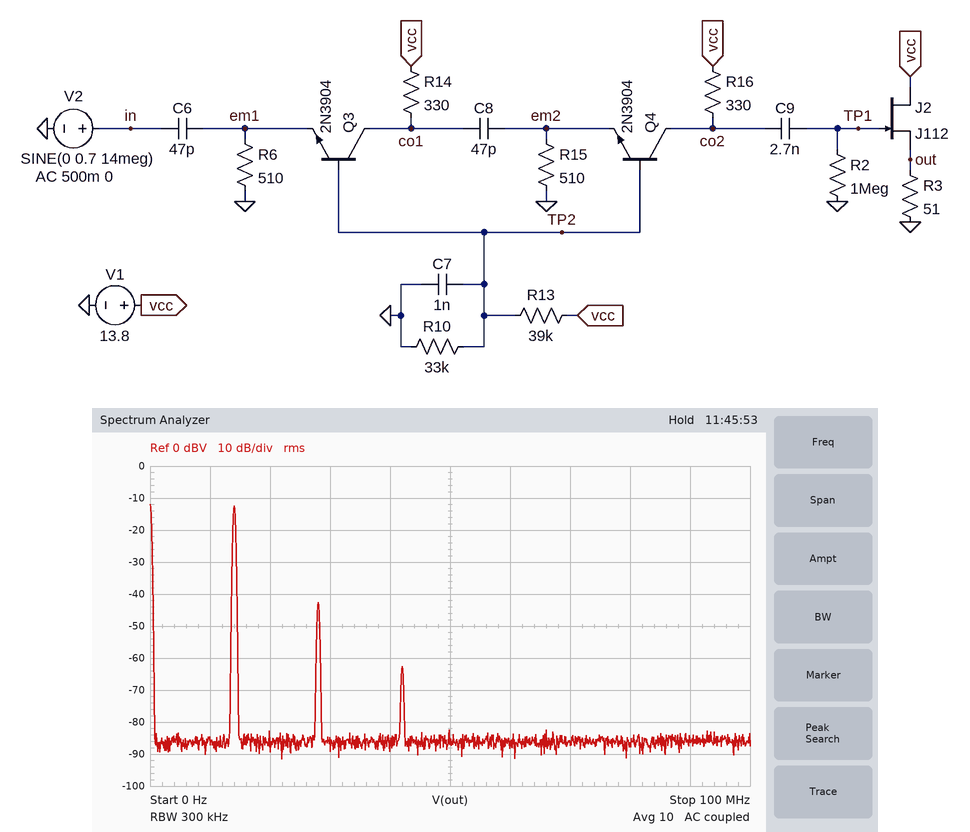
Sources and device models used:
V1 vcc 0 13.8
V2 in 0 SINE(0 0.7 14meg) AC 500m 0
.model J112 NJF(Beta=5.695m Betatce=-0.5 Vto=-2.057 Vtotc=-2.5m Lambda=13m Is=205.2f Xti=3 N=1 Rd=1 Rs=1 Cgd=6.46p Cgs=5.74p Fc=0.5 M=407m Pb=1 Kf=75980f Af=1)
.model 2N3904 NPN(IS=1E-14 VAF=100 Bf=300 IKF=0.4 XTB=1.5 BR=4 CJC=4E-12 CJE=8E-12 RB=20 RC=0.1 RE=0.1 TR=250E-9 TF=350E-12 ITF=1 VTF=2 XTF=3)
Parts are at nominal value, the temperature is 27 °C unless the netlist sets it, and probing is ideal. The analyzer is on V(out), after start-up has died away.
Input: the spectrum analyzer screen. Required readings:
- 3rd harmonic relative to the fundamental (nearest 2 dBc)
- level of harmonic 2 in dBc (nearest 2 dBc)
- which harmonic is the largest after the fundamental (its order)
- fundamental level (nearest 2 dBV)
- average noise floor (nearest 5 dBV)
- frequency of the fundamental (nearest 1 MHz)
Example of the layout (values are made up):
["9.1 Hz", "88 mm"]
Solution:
["-50 dBc", "-30 dBc", "2", "-12 dBV", "-85 dBV", "14 MHz"]
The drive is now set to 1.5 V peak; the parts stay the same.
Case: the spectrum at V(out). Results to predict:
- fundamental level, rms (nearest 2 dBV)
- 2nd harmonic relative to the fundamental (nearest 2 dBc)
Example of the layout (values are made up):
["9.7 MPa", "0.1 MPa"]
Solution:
["-6 dBV", "-22 dBc"]
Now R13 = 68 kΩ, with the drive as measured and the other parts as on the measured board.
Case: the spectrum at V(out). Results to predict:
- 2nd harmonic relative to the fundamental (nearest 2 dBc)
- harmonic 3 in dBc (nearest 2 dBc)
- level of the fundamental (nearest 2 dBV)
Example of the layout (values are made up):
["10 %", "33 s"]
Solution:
["-32 dBc", "-46 dBc", "-12 dBV"]
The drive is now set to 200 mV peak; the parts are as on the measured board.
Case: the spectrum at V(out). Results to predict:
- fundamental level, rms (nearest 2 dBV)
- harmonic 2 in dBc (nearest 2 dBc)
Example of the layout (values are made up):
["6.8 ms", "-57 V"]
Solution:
["-24 dBV", "-42 dBc"]
